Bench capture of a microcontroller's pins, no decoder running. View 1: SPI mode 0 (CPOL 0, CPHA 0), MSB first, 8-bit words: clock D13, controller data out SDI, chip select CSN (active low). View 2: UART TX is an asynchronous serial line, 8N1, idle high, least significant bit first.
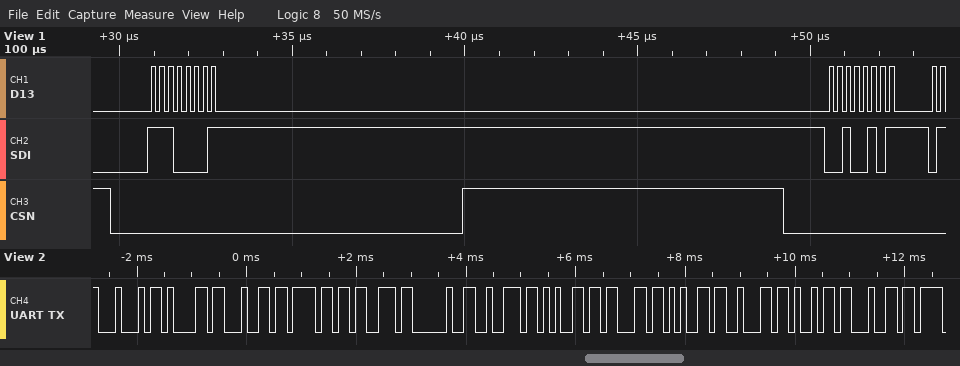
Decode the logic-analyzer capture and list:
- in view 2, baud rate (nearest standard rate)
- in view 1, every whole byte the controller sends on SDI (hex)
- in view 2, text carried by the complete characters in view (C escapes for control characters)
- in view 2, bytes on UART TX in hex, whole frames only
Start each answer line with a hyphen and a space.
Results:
- 9600 baud
- 0xE1 0x25
- "Dados recebid"
- 0x44 0x61 0x64 0x6F 0x73 0x20 0x72 0x65 0x63 0x65 0x62 0x69 0x64
